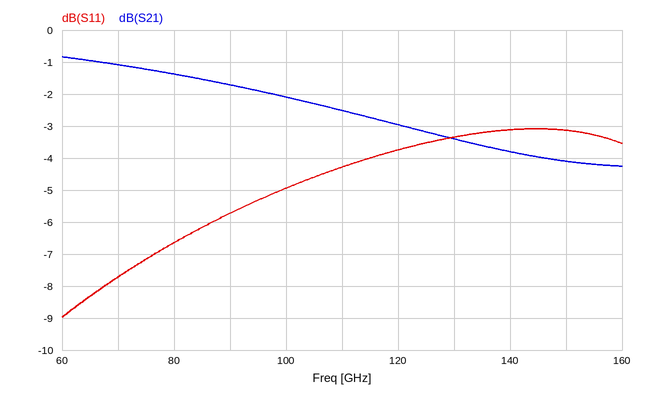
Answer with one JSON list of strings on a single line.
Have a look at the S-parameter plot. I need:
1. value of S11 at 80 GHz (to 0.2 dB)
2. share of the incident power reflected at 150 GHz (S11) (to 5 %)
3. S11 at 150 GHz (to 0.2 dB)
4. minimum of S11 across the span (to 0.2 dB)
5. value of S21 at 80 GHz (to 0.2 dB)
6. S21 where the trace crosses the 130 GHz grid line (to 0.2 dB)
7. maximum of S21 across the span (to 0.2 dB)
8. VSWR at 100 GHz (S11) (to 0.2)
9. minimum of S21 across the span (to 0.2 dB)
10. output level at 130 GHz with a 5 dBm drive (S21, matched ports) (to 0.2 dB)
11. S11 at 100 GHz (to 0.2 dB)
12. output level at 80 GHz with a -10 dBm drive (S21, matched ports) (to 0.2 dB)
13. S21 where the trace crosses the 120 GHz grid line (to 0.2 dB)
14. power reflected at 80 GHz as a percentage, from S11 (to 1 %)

["-6.6 dB", "50 %", "-3.2 dB", "-9.0 dB", "-1.4 dB", "-3.4 dB", "-0.8 dB", "3.6", "-4.2 dB", "1.6 dBm", "-5.0 dB", "-11.4 dBm", "-3.0 dB", "22 %"]
